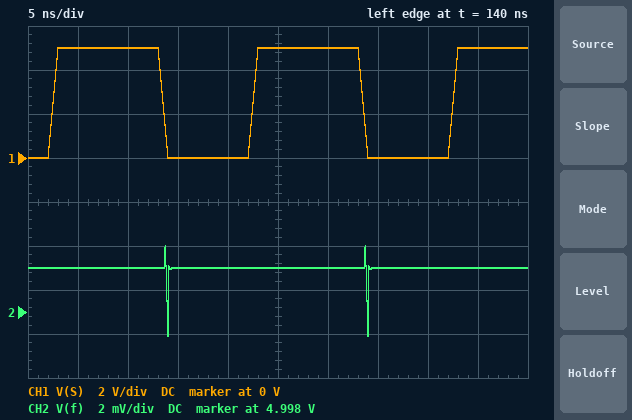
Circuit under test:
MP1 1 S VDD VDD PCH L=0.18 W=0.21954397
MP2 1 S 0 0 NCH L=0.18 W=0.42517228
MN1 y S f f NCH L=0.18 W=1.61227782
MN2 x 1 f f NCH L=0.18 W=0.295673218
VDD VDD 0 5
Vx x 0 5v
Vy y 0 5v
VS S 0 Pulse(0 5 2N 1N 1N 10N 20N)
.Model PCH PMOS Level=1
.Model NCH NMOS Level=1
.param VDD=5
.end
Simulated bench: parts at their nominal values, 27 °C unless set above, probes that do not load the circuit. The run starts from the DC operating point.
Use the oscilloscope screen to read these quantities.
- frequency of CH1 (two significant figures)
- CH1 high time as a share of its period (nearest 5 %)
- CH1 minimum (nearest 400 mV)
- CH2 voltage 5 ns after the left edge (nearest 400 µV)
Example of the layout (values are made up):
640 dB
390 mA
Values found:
50 MHz
55 %
0 V
5.0000 V
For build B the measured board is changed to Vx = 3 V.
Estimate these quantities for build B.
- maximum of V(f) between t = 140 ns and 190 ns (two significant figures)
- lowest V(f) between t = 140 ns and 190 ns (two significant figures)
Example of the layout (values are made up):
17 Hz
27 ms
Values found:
3.6 V
3.0 V
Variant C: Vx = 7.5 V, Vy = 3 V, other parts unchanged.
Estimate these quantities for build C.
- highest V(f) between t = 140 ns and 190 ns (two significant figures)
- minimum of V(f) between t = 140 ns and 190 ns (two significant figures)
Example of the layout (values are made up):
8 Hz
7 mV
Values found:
3.6 V
3.0 V
